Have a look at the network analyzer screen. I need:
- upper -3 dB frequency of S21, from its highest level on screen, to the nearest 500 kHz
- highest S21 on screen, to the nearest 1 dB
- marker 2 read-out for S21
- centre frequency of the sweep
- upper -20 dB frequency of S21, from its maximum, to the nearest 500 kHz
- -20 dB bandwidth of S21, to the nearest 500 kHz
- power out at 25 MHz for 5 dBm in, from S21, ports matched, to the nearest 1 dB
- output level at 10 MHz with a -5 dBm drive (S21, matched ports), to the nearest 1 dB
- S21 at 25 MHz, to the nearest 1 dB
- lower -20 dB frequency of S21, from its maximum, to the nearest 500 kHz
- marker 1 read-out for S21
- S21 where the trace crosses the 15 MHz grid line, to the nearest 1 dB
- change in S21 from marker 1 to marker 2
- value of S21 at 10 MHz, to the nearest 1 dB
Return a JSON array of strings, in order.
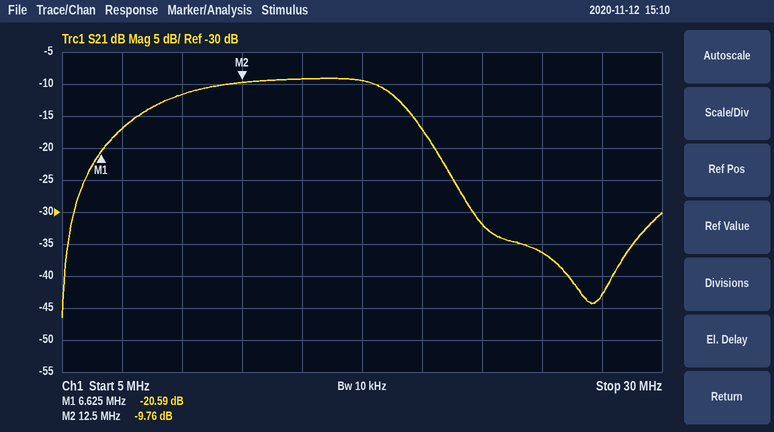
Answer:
["19.0 MHz", "-9 dB", "-9.76 dB", "17.5 MHz", "22.0 MHz", "16.5 MHz", "-31 dBm", "-17 dBm", "-36 dB", "5.5 MHz", "-20.59 dB", "-9 dB", "10.83 dB", "-12 dB"]
